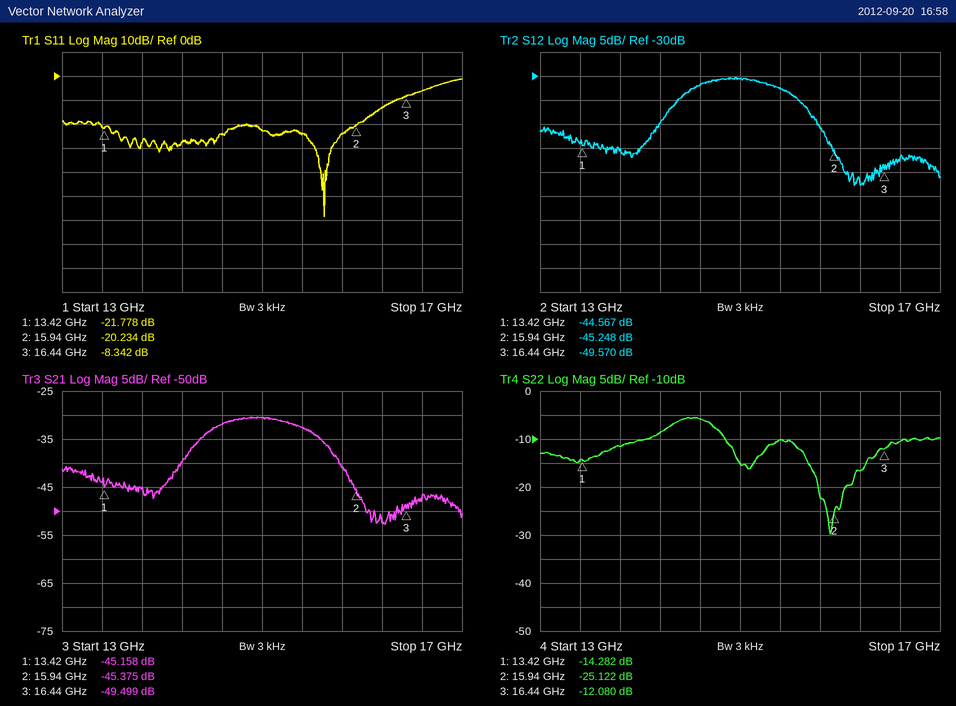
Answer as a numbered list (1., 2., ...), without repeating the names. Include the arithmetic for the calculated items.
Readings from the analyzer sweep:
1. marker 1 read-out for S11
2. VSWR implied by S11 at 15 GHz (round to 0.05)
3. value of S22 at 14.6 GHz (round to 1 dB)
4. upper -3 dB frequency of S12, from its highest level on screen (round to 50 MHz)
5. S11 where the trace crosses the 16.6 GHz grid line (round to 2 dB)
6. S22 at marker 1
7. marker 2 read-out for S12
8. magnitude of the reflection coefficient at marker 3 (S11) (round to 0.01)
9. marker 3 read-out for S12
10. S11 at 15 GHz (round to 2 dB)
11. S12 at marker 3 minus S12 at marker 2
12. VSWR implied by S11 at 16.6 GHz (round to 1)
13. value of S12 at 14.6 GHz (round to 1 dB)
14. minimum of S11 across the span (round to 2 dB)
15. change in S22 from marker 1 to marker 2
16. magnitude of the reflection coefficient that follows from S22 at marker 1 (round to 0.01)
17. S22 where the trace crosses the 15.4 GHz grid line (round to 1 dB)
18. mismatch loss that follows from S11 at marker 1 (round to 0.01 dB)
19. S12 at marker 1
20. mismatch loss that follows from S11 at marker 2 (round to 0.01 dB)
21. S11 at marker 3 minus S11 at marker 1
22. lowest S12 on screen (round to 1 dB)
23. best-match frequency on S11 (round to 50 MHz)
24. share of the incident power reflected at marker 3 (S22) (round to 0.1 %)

1. -21.778 dB
2. |Γ| = 10^(-22/20) = 0.0794; VSWR = (1 + 0.0794)/(1 − 0.0794) ≈ 1.17, so 1.15 to the nearest 0.05
3. -6 dB
4. 15.50 GHz
5. -6 dB
6. -14.282 dB
7. -45.248 dB
8. 10^(-8.342/20) ≈ 0.38
9. -49.570 dB
10. -22 dB
11. -49.57 − (-45.248) = -4.322 dB
12. |Γ| = 10^(-6/20) = 0.5012; VSWR = (1 + 0.5012)/(1 − 0.5012) ≈ 3
13. -32 dB
14. -58 dB
15. -25.122 − (-14.282) = -10.840 dB
16. 10^(-14.282/20) ≈ 0.19
17. -10 dB
18. −10 log10(1 − 10^(-21.778/10)) ≈ 0.03 dB
19. -44.567 dB
20. −10 log10(1 − 10^(-20.234/10)) ≈ 0.04 dB
21. -8.342 − (-21.778) = 13.436 dB
22. -53 dB
23. 15.60 GHz
24. 10^(-12.08/10) ≈ 6.2 %
